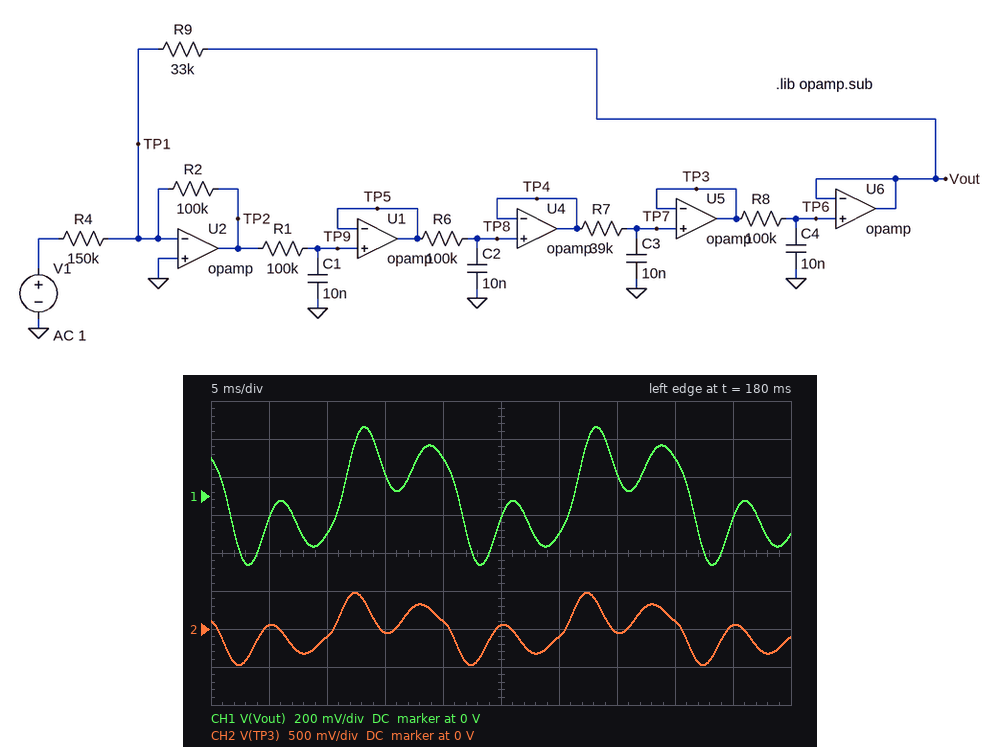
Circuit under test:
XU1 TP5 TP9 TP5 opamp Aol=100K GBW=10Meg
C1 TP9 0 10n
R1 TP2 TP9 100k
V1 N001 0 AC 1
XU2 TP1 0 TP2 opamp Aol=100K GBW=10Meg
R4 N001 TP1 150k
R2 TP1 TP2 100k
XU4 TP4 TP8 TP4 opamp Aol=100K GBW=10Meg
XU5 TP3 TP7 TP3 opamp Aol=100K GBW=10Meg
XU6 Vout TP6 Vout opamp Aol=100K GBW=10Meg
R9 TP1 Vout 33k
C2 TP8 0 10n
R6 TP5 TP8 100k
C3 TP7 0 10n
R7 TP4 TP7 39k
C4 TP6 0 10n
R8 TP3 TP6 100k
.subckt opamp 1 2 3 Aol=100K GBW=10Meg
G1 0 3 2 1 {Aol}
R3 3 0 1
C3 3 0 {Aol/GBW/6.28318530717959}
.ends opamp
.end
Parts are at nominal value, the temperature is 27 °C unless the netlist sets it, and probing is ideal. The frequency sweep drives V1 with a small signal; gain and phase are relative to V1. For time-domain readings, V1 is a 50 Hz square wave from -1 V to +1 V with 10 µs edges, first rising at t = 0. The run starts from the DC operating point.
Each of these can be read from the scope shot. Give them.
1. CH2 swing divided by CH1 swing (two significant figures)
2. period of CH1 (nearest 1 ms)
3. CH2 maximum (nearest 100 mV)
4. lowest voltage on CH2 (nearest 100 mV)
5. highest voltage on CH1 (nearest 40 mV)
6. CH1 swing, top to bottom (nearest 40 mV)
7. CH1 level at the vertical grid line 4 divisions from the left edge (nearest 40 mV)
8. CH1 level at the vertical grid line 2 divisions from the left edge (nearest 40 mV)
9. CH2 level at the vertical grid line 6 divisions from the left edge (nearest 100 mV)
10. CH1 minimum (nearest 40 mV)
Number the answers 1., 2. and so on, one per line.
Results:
1. 1.3
2. 20 ms
3. 500 mV
4. -500 mV
5. 360 mV
6. 720 mV
7. 200 mV
8. -200 mV
9. -100 mV
10. -360 mV
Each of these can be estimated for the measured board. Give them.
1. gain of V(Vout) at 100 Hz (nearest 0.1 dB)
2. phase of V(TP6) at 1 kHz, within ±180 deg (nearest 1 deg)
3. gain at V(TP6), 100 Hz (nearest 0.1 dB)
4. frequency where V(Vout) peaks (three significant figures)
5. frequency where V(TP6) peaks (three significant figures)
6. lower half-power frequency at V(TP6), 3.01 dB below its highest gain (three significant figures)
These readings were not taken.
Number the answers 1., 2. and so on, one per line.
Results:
1. -12.8 dB
2. -131 deg
3. -12.8 dB
4. 177 Hz
5. 177 Hz
6. 156 Hz
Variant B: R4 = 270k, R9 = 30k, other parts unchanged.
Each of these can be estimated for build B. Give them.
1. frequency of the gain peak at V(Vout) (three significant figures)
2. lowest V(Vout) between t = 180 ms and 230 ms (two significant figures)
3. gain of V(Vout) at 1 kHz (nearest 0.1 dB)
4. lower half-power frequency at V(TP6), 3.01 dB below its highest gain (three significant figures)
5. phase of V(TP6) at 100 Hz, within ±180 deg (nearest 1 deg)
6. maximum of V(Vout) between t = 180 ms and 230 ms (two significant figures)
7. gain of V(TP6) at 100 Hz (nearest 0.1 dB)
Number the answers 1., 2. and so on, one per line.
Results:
1. 182 Hz
2. -180 mV
3. -65.3 dB
4. 166 Hz
5. 150 deg
6. 180 mV
7. -18.7 dB
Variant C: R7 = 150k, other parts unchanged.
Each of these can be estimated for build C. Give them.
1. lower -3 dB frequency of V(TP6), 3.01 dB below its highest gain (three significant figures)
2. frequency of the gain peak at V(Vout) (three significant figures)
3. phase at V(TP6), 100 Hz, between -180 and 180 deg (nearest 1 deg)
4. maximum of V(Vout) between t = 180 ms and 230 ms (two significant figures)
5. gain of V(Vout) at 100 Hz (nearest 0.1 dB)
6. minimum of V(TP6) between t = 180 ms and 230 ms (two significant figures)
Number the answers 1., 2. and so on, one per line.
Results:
1. 121 Hz
2. 132 Hz
3. 132 deg
4. 410 mV
5. -9.4 dB
6. -410 mV
